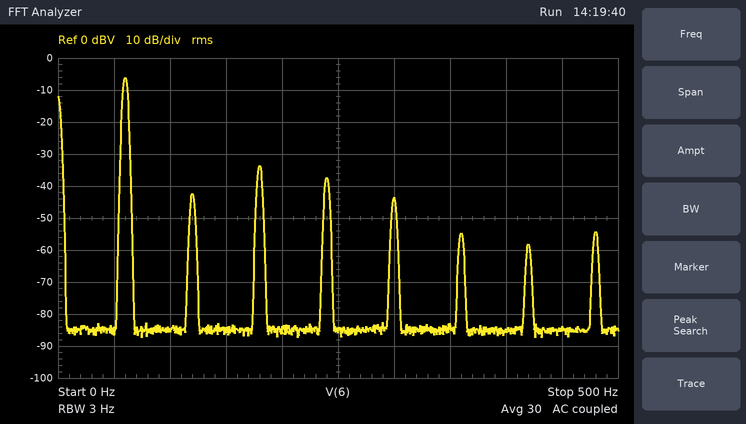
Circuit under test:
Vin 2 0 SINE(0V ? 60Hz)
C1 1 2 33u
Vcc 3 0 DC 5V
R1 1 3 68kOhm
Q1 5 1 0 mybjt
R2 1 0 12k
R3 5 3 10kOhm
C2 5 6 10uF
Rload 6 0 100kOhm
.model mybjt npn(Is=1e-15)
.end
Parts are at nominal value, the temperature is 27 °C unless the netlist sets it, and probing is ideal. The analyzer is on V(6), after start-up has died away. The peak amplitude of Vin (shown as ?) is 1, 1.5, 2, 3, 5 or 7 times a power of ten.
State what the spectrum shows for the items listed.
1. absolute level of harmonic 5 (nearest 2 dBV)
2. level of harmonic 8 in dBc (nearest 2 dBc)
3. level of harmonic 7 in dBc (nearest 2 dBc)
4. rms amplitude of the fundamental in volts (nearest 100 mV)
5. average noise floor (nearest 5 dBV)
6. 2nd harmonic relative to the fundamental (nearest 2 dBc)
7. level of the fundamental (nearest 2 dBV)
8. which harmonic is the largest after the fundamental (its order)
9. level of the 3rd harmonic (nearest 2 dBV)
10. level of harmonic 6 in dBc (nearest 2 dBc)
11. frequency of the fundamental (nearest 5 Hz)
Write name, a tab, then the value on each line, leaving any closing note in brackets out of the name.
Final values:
absolute level of harmonic 5	-44 dBV
level of harmonic 8 in dBc	-48 dBc
level of harmonic 7 in dBc	-52 dBc
rms amplitude of the fundamental in volts	500 mV
average noise floor	-85 dBV
2nd harmonic relative to the fundamental	-36 dBc
level of the fundamental	-6 dBV
which harmonic is the largest after the fundamental	3
level of the 3rd harmonic	-34 dBV
level of harmonic 6 in dBc	-48 dBc
frequency of the fundamental	60 Hz
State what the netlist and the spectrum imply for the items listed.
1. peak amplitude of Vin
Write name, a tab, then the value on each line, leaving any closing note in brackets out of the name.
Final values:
peak amplitude of Vin	5 mV
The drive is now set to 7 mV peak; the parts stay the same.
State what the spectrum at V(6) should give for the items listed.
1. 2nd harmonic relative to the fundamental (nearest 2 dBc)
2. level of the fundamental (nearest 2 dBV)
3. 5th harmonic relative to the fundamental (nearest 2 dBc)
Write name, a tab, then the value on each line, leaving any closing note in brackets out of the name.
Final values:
2nd harmonic relative to the fundamental	-34 dBc
level of the fundamental	-4 dBV
5th harmonic relative to the fundamental	-36 dBc
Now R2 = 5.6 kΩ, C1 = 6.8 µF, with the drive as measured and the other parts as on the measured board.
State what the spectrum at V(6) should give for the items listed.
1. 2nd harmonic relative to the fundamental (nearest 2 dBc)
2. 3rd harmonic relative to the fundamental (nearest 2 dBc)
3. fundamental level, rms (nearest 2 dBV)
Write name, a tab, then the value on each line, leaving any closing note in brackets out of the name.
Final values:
2nd harmonic relative to the fundamental	-26 dBc
3rd harmonic relative to the fundamental	-56 dBc
fundamental level, rms	-110 dBV
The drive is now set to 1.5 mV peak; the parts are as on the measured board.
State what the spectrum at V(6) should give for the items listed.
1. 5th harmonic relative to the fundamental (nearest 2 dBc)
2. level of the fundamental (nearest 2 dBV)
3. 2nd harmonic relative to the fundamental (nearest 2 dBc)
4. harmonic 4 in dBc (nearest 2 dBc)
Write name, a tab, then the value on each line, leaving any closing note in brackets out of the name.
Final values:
5th harmonic relative to the fundamental	-54 dBc
level of the fundamental	-16 dBV
2nd harmonic relative to the fundamental	-24 dBc
harmonic 4 in dBc	-36 dBc
